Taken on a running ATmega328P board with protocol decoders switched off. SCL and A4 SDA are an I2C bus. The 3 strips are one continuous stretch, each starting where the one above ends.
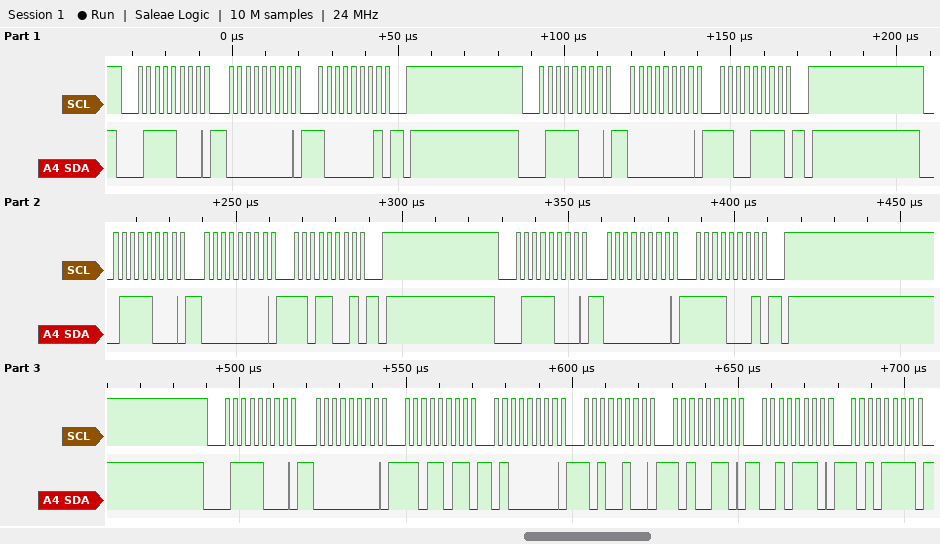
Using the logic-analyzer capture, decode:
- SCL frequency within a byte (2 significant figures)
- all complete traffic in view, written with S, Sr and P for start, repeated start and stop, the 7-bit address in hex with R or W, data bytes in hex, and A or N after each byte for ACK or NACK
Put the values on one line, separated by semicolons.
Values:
400 kHz; S 3CW A 00 A 81 A P S 3CW A 00 A CF A P S 3CW A 00 A D9 A P S 3CW A 00 A F1 A P S 3CW A 00 A DB A 40 A A4 A A6 A 2E A AF A
